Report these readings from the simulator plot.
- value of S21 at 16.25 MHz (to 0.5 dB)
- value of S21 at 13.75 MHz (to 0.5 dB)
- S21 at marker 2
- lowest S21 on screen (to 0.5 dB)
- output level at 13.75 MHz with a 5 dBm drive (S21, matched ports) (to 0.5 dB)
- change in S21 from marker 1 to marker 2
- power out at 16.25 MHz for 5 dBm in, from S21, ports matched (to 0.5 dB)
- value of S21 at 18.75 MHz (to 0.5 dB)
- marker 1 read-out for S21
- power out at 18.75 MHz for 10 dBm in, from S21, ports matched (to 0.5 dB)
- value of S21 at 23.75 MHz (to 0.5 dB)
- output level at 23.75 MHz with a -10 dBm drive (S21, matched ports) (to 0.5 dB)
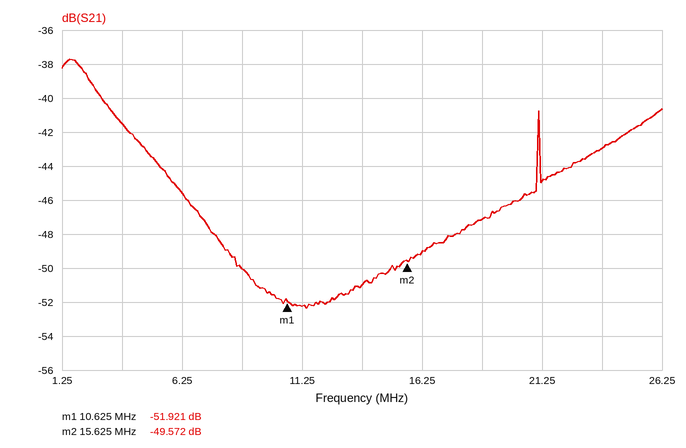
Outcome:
-49.0 dB
-51.0 dB
-49.572 dB
-52.5 dB
-46.0 dBm
2.349 dB
-44.0 dBm
-47.0 dB
-51.921 dB
-37.0 dBm
-43.0 dB
-53.0 dBm
